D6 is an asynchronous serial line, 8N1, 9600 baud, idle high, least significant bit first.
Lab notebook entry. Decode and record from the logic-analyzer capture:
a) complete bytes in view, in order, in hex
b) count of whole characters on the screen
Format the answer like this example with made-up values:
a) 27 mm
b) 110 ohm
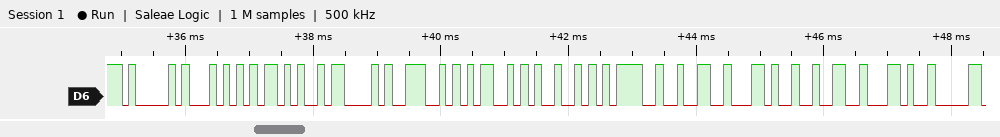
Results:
a) 0x41 0x54 0x2B 0x43 0x4E 0x4D 0x49 0x3D 0x32 0x2C 0x32 0x2C
b) 12
